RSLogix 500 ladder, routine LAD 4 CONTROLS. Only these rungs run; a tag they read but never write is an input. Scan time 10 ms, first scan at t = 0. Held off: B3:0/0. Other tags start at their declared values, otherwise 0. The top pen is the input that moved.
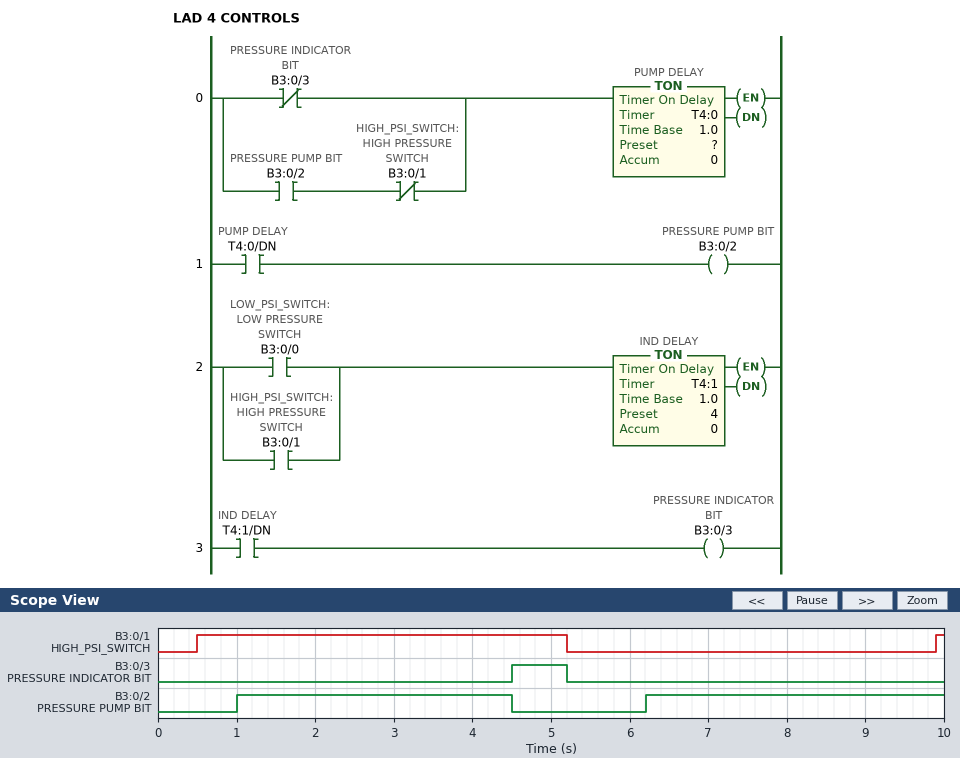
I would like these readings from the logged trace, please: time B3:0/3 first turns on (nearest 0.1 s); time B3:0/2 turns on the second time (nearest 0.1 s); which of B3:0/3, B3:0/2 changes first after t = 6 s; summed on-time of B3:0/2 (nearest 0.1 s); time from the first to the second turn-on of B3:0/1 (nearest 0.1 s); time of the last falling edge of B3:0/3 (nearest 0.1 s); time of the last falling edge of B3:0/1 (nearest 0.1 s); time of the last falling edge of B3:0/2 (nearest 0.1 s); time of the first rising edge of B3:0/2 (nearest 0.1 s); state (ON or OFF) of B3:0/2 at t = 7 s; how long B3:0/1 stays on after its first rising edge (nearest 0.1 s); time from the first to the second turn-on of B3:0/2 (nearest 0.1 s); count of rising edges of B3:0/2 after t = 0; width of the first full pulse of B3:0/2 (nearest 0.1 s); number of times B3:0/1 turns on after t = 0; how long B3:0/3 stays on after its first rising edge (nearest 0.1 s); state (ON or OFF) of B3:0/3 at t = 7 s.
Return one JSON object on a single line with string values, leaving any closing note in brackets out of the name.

{"time B3:0/3 first turns on": "4.5 s", "time B3:0/2 turns on the second time": "6.2 s", "which of B3:0/3, B3:0/2 changes first after t = 6 s": "B3:0/2", "summed on-time of B3:0/2": "7.3 s", "time from the first to the second turn-on of B3:0/1": "9.4 s", "time of the last falling edge of B3:0/3": "5.2 s", "time of the last falling edge of B3:0/1": "5.2 s", "time of the last falling edge of B3:0/2": "4.5 s", "time of the first rising edge of B3:0/2": "1.0 s", "state (ON or OFF) of B3:0/2 at t = 7 s": "ON", "how long B3:0/1 stays on after its first rising edge": "4.7 s", "time from the first to the second turn-on of B3:0/2": "5.2 s", "count of rising edges of B3:0/2 after t = 0": "2", "width of the first full pulse of B3:0/2": "3.5 s", "number of times B3:0/1 turns on after t = 0": "2", "how long B3:0/3 stays on after its first rising edge": "0.7 s", "state (ON or OFF) of B3:0/3 at t = 7 s": "OFF"}
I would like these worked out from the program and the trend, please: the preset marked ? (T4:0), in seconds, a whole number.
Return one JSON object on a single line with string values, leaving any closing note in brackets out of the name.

{"the preset marked ? (T4:0), in seconds, a whole number": "1 s"}
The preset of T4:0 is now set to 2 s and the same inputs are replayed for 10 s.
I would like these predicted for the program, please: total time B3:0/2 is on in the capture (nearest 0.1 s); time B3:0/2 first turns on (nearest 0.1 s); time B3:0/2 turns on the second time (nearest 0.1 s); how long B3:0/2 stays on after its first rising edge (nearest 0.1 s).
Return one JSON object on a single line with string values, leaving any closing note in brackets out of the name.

{"total time B3:0/2 is on in the capture": "5.3 s", "time B3:0/2 first turns on": "2.0 s", "time B3:0/2 turns on the second time": "7.2 s", "how long B3:0/2 stays on after its first rising edge": "2.5 s"}
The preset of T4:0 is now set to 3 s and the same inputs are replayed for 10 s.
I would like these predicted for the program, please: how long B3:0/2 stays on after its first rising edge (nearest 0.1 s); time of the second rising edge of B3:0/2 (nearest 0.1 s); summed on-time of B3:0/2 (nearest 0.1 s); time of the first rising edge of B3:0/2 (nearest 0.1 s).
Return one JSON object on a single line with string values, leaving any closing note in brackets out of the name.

{"how long B3:0/2 stays on after its first rising edge": "1.5 s", "time of the second rising edge of B3:0/2": "8.2 s", "summed on-time of B3:0/2": "3.3 s", "time of the first rising edge of B3:0/2": "3.0 s"}
